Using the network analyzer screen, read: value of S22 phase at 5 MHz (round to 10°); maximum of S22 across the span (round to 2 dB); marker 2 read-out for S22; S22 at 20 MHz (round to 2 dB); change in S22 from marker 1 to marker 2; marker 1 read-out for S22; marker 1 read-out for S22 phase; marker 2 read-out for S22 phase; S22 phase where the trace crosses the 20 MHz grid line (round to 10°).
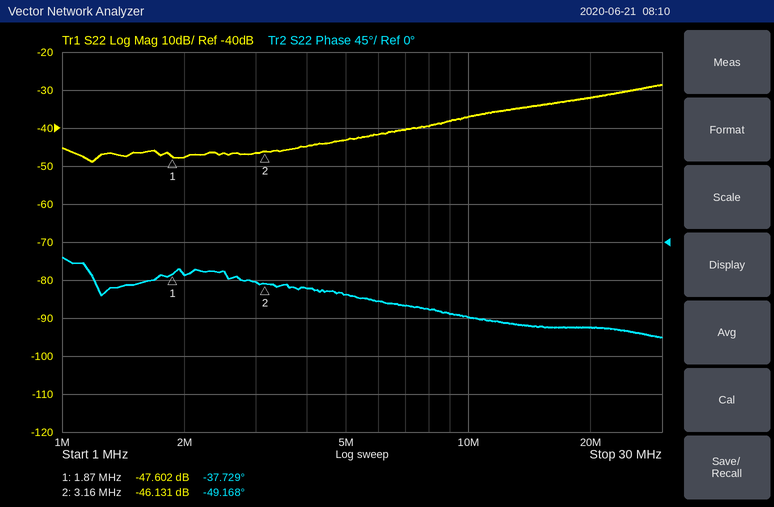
-60°
-28 dB
-46.131 dB
-32 dB
1.471 dB
-47.602 dB
-37.729°
-49.168°
-100°
